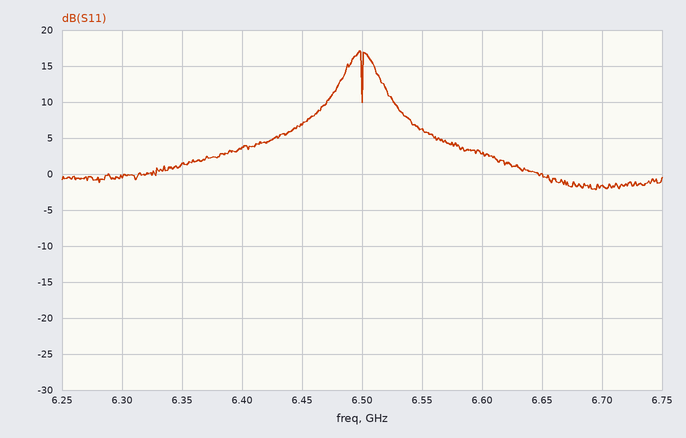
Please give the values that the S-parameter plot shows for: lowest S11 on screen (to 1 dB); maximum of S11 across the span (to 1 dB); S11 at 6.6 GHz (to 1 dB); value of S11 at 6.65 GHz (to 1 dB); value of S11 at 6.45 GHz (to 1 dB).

-2 dB
17 dB
3 dB
0 dB
7 dB
